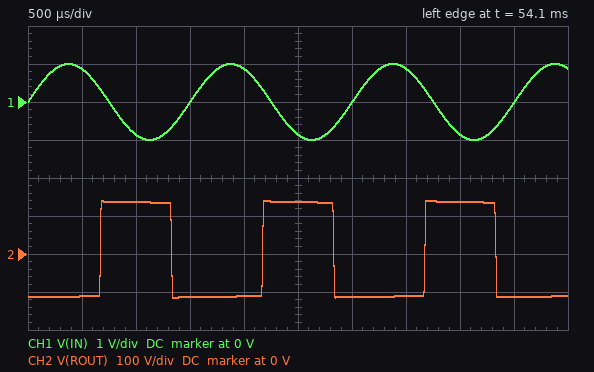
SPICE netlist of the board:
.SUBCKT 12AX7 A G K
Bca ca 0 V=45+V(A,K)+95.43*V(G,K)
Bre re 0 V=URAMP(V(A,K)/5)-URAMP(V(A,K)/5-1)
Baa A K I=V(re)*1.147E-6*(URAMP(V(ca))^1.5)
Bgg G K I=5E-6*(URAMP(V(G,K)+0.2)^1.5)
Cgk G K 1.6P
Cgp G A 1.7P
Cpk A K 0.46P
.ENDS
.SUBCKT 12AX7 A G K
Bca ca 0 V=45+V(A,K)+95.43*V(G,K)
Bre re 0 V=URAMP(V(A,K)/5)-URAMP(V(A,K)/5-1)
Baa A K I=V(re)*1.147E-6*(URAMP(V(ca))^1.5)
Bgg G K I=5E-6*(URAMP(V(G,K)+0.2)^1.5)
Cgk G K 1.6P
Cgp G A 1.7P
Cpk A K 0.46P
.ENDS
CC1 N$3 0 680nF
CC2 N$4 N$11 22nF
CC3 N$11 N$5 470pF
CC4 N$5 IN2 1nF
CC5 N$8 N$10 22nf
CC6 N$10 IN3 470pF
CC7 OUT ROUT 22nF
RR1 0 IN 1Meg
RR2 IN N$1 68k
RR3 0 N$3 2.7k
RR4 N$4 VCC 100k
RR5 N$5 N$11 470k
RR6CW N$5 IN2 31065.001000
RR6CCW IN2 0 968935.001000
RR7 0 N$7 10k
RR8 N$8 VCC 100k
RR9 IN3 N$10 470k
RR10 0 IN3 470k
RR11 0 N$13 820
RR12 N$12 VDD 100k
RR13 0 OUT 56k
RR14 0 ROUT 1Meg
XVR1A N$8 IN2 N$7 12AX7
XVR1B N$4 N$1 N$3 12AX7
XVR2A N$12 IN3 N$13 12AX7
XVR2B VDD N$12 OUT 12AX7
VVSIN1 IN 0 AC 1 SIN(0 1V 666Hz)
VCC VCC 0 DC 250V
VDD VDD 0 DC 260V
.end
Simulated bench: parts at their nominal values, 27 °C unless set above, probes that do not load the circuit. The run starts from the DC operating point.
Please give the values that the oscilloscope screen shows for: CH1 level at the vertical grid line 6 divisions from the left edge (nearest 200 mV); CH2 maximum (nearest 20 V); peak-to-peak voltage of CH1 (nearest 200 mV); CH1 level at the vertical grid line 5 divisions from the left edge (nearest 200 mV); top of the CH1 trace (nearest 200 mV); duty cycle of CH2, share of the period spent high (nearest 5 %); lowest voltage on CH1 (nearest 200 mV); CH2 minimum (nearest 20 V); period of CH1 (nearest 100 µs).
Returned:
0 V
140 V
2.0 V
-800 mV
1.0 V
45 %
-1.0 V
-120 V
1.5 ms
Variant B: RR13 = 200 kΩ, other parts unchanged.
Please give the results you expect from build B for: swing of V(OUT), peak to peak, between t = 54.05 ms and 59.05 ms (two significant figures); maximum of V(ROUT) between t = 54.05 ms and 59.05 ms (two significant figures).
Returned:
240 V
130 V
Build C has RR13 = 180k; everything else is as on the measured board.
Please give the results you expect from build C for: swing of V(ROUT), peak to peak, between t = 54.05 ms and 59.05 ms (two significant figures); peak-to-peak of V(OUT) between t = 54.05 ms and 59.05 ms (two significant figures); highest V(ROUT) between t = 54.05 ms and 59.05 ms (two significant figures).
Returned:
250 V
240 V
130 V
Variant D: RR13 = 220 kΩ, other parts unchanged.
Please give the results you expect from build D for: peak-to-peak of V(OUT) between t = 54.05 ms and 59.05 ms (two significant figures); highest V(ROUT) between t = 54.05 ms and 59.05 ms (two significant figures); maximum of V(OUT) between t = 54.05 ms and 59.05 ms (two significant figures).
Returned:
240 V
130 V
260 V
